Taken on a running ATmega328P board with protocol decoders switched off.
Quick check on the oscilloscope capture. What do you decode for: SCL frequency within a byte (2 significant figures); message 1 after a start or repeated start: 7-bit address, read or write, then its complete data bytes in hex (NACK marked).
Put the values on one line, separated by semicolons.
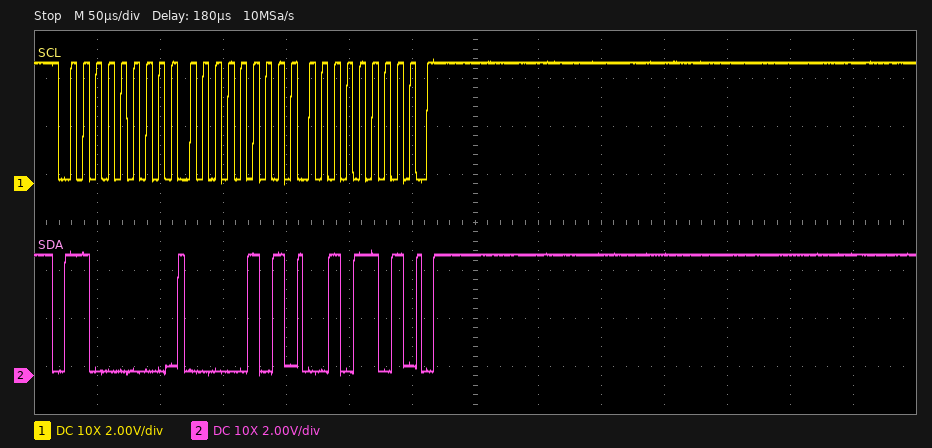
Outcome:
100 kHz; 0x60 write: 05 2D
